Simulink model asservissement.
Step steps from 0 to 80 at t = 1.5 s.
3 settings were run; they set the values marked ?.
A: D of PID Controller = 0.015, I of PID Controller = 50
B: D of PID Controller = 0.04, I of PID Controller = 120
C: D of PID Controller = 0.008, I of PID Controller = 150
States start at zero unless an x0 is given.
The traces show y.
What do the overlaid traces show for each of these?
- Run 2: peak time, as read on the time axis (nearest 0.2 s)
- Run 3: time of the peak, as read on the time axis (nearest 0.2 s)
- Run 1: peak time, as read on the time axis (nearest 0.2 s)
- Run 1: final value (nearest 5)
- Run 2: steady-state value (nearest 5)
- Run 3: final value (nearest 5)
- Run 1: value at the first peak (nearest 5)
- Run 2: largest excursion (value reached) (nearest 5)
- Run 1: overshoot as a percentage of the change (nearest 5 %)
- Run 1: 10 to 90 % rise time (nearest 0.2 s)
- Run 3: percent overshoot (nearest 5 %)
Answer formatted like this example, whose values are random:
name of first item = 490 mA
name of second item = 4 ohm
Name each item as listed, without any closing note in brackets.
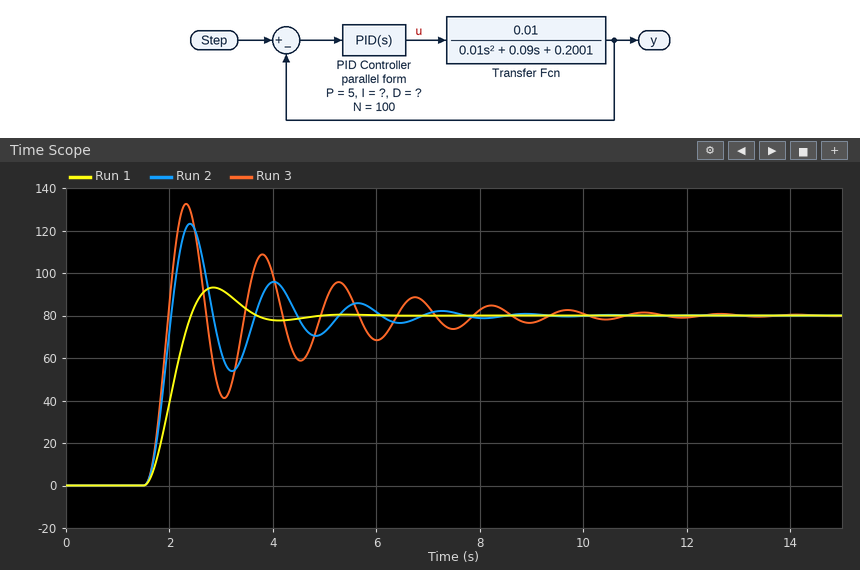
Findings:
Run 2: peak time, as read on the time axis = 2.4 s
Run 3: time of the peak, as read on the time axis = 2.4 s
Run 1: peak time, as read on the time axis = 2.8 s
Run 1: final value = 80
Run 2: steady-state value = 80
Run 3: final value = 80
Run 1: value at the first peak = 95
Run 2: largest excursion (value reached) = 125
Run 1: overshoot as a percentage of the change = 15 %
Run 1: 10 to 90 % rise time = 0.6 s
Run 3: percent overshoot = 65 %
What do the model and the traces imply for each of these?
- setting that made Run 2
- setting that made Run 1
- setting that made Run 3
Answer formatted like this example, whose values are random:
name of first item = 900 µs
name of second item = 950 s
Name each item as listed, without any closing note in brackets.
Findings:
setting that made Run 2 = B
setting that made Run 1 = A
setting that made Run 3 = C
